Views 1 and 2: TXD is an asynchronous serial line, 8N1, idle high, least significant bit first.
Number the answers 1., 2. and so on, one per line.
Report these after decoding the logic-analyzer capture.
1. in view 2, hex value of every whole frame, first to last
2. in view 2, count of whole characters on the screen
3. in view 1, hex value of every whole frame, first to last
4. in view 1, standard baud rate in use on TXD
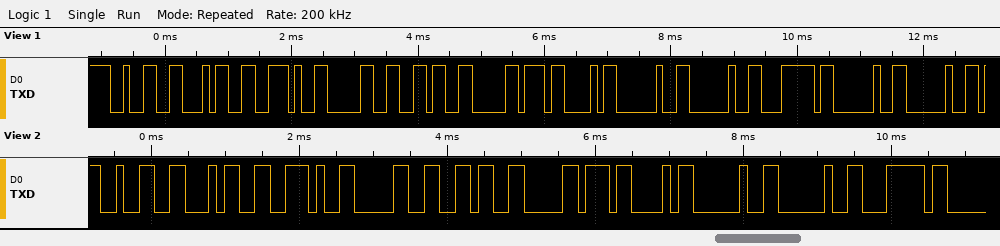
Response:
1. 0x32 0x34 0x2E 0x30 0x36 0xB0 0x43 0x20 0x20 0x7C
2. 10
3. 32 34 2E 30 36 B0 43 20 20 7C 20 20
4. 9600 baud
